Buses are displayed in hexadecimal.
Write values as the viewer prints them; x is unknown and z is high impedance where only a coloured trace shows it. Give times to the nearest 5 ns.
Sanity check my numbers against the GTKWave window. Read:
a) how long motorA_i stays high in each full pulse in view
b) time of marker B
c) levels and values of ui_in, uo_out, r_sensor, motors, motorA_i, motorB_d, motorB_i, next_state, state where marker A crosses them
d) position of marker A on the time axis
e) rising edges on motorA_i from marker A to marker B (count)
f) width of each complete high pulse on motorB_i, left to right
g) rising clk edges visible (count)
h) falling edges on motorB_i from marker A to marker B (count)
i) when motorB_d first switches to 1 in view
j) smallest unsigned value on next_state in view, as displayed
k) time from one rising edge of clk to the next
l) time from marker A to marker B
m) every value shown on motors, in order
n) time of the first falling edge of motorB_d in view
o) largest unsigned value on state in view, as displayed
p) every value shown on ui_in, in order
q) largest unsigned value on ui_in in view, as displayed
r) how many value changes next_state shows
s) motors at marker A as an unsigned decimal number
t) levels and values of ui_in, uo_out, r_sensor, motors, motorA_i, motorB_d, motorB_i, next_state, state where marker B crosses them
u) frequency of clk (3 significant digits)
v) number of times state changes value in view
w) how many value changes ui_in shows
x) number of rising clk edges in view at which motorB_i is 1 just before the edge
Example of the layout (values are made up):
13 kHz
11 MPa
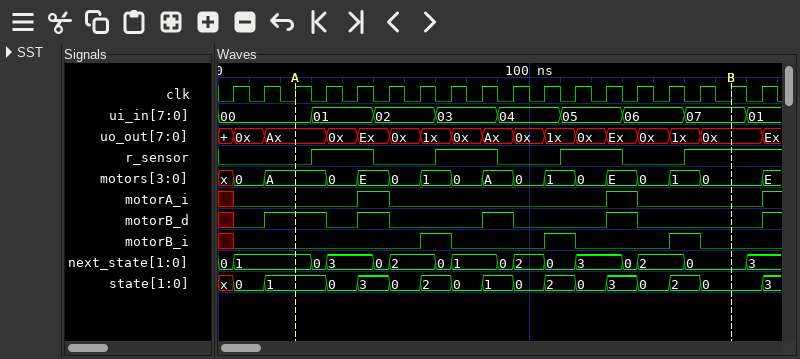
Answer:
10 ns, 10 ns
165 ns
ui_in=00, uo_out=Ax, r_sensor=0, motors=A, motorA_i=0, motorB_d=1, motorB_i=0, next_state=1, state=1
25 ns
2
10 ns, 10 ns, 10 ns
18
3
15 ns
0
10 ns
140 ns
x, 0, A, 0, E, 0, 1, 0, A, 0, 1, 0, E, 0, 1, 0, E
35 ns
3
00, 01, 02, 03, 04, 05, 06, 07, 01
07
15
10
ui_in=07, uo_out=0x, r_sensor=1, motors=0, motorA_i=0, motorB_d=0, motorB_i=0, next_state=0, state=0
100 MHz
16
8
3
